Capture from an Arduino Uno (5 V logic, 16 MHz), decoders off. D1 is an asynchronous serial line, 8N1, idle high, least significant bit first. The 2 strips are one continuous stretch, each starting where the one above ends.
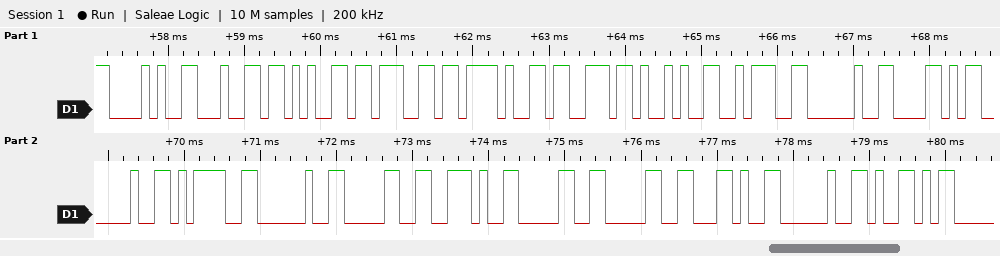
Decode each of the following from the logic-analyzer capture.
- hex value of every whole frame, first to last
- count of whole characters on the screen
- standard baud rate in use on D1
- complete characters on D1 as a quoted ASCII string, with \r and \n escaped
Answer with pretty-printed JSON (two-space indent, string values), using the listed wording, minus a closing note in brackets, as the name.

{
  "hex value of every whole frame, first to last": "28 64 65 67 2F 73 29 3A 20 58 20 3D 20 30 2E 30 30 2C 20 59",
  "count of whole characters on the screen": "20",
  "standard baud rate in use on D1": "9600 baud",
  "complete characters on D1 as a quoted ASCII string, with \\r and \\n escaped": "\"(deg/s): X = 0.00, Y\""
}
